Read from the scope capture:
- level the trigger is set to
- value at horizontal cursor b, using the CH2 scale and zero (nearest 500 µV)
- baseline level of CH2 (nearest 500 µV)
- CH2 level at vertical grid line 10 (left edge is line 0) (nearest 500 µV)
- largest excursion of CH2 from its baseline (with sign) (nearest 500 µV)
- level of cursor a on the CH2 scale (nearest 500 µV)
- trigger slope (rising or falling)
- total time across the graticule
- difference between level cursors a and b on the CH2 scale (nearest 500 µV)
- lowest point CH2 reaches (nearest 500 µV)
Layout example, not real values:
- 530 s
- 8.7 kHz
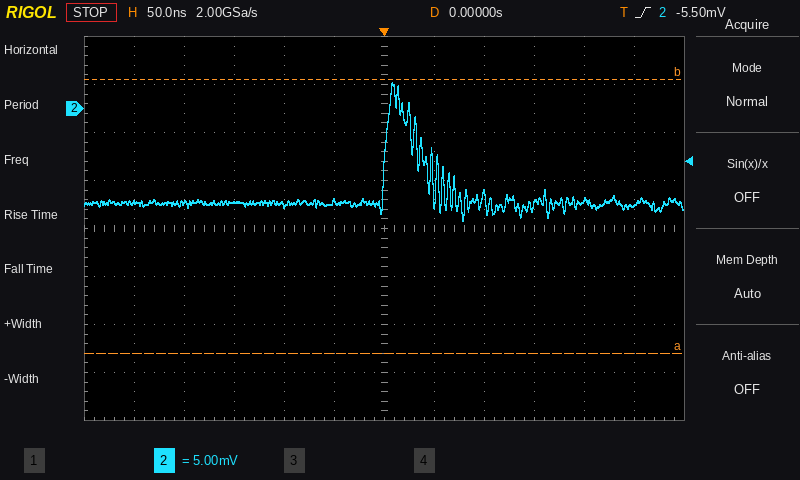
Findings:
- -5.50 mV
- 3.0 mV
- -10.0 mV
- -9.5 mV
- +12.5 mV
- -25.5 mV
- rising
- 600 ns
- 28.5 mV
- -11.5 mV
